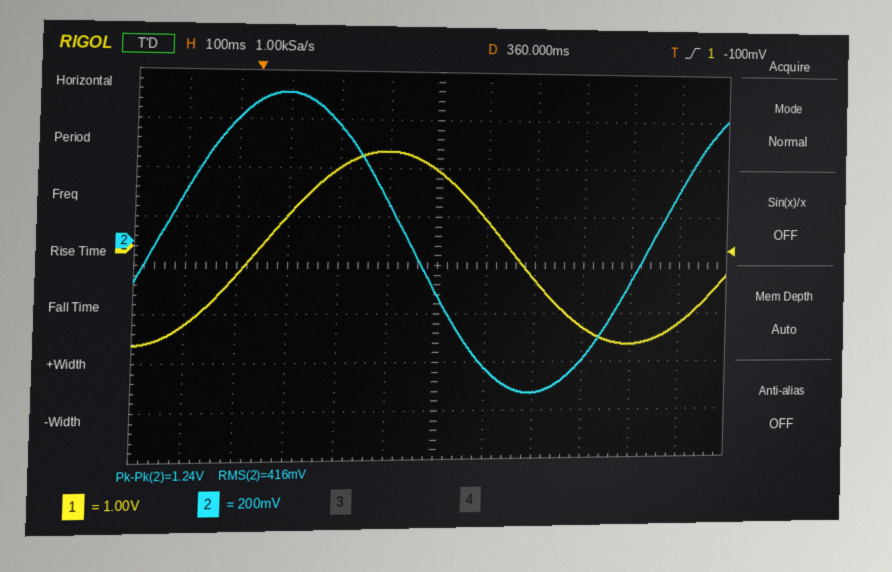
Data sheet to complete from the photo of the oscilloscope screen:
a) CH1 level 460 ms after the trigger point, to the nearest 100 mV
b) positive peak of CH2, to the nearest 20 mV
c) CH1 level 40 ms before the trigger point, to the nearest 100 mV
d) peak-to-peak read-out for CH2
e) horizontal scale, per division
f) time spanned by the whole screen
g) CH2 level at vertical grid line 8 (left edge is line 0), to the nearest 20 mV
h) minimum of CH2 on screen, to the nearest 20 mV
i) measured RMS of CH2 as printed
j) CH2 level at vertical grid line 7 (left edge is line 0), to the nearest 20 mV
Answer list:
500 mV
620 mV
-600 mV
1.24 V
100 ms
1.2 s
-620 mV
-620 mV
416 mV
-520 mV
